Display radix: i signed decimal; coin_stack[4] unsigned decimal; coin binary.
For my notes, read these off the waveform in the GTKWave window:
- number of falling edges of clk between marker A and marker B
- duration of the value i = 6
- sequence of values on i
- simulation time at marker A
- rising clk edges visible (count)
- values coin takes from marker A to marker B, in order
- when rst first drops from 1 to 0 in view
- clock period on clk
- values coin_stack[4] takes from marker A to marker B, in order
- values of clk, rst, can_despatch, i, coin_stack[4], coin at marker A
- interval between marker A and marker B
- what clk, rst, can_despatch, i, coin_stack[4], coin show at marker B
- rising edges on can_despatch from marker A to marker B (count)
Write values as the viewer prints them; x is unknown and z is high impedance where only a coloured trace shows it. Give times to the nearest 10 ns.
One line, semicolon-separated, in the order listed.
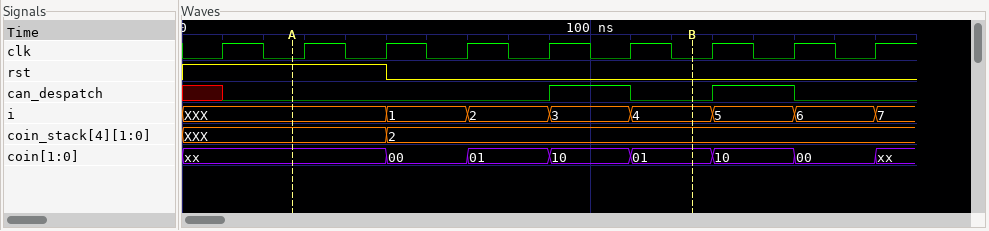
5; 20 ns; XXX, 1, 2, 3, 4, 5, 6, 7; 30 ns; 9; xx, 00, 01, 10, 01; 50 ns; 20 ns; XXX, 2; clk=0, rst=1, can_despatch=0, i=XXX, coin_stack[4]=XXX, coin=xx; 100 ns; clk=0, rst=0, can_despatch=0, i=4, coin_stack[4]=2, coin=01; 1
